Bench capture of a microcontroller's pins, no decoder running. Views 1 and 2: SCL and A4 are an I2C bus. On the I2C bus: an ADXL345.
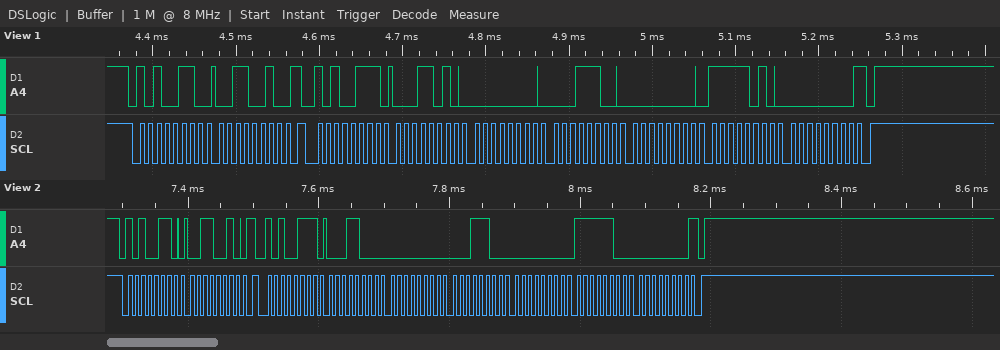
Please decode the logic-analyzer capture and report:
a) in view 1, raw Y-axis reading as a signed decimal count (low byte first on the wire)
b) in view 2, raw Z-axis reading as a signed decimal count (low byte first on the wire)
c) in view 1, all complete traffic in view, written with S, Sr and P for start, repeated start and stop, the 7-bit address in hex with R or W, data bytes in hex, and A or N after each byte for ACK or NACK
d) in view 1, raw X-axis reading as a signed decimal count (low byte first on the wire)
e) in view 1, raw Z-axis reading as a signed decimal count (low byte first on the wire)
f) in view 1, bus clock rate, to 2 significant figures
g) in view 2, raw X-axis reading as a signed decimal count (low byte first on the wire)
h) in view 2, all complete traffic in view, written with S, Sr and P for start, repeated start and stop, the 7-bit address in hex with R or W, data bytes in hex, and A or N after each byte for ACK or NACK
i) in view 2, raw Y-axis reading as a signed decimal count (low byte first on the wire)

28
252
S 53W A 32 A Sr 53R A 1A A 00 A 1C A 00 A FA A 00 N P
26
250
100 kHz
24
S 53W A 32 A Sr 53R A 18 A 00 A 1C A 00 A FC A 00 N P
28
